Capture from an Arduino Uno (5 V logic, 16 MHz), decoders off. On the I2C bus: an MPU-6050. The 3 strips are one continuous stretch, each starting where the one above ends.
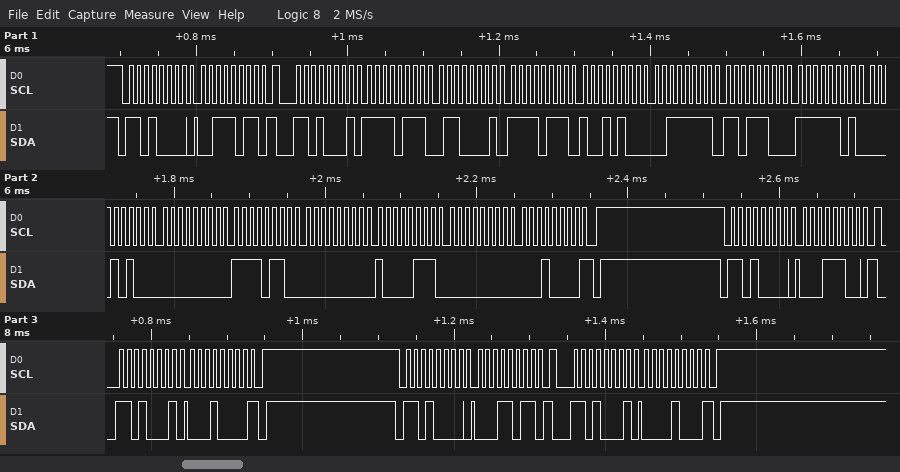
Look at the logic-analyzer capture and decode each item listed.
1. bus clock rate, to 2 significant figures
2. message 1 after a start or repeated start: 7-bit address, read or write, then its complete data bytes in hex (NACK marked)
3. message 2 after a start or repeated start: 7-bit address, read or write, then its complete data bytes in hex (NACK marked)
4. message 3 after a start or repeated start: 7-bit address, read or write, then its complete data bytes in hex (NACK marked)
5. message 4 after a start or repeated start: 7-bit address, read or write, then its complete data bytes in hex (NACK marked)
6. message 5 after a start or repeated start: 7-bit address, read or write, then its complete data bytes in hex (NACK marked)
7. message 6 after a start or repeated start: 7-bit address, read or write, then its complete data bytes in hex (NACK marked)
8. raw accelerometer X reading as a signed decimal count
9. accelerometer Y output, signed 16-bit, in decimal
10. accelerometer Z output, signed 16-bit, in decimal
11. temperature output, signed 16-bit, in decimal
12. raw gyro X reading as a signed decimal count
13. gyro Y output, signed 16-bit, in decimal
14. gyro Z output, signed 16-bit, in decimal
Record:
100 kHz
0x68 write: 3B
0x68 read: F7 61 F7 94 3F DC FD 14 00 F6 00 87 00 10 NACK
0x68 write: 1C
0x68 read: 10 NACK
0x68 write: 1B
0x68 read: 08 NACK
-2207
-2156
16348
-748
246
135
16
